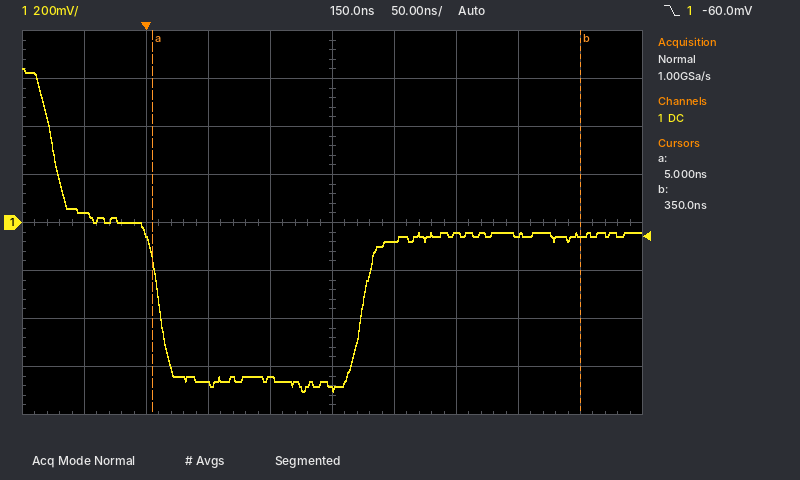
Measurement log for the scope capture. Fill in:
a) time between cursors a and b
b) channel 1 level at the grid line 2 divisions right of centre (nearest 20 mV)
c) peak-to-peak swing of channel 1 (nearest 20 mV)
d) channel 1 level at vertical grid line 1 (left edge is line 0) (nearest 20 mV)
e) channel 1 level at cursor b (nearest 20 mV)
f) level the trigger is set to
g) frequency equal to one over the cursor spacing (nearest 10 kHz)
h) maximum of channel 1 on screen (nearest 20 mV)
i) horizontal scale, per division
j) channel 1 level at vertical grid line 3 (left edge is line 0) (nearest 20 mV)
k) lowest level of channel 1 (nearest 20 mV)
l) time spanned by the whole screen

345 ns
-40 mV
1.34 V
40 mV
-60 mV
-60.0 mV
2.90 MHz
640 mV
50 ns
-680 mV
-700 mV
500 ns
